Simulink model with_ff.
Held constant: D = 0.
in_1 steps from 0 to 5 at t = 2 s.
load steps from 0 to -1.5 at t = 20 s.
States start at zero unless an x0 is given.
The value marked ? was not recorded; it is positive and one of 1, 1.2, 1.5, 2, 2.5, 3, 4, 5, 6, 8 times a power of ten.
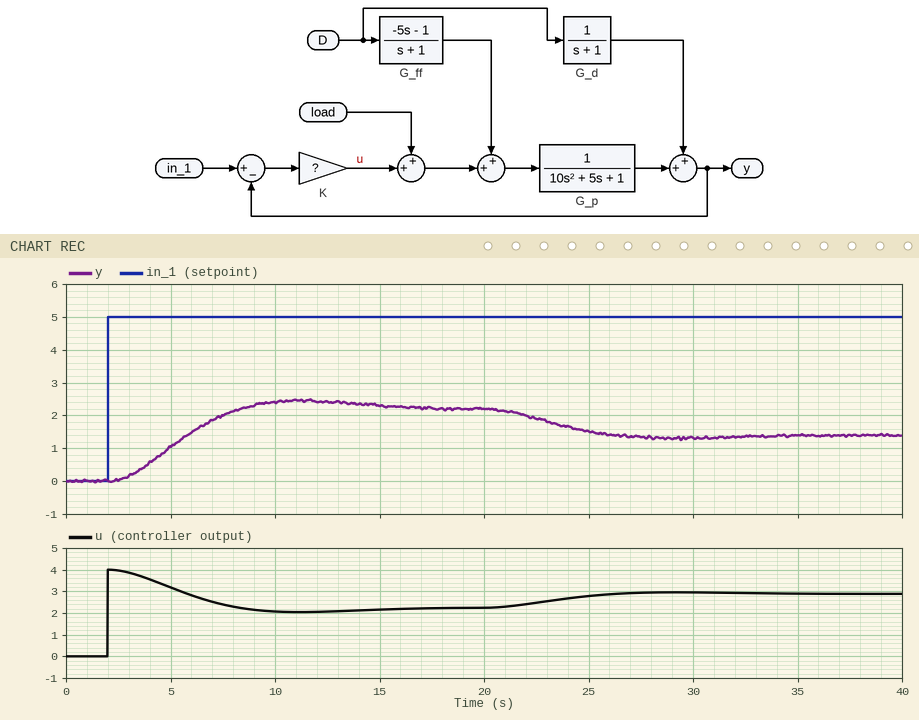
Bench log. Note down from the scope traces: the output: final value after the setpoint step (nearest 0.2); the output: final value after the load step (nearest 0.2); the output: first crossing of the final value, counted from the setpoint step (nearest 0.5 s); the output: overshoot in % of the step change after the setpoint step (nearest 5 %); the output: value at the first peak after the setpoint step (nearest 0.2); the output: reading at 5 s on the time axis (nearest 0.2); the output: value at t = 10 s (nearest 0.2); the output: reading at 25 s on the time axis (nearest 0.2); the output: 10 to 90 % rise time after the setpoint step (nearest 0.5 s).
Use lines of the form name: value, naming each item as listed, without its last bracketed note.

the output: final value after the setpoint step: 2.2
the output: final value after the load step: 1.4
the output: first crossing of the final value, counted from the setpoint step: 6.5 s
the output: overshoot in % of the step change after the setpoint step: 10 %
the output: value at the first peak after the setpoint step: 2.4
the output: reading at 5 s on the time axis: 1.0
the output: value at t = 10 s: 2.4
the output: reading at 25 s on the time axis: 1.6
the output: 10 to 90 % rise time after the setpoint step: 4.5 s
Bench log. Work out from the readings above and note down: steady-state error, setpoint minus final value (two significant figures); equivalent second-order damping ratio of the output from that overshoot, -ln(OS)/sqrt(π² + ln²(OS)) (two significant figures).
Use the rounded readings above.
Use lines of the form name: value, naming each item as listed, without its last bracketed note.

steady-state error, setpoint minus final value: 2.8
equivalent second-order damping ratio of the output from that overshoot, -ln(OS)/sqrt(π² + ln²(OS)): 0.59
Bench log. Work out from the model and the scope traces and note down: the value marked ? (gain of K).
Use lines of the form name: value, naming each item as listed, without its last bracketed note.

the value marked ?: 0.8
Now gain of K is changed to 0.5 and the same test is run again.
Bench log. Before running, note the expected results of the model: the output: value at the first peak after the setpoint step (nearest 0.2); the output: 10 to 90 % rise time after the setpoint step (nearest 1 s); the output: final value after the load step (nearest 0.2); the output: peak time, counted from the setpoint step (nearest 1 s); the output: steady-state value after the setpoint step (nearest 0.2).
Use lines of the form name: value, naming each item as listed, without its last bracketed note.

the output: value at the first peak after the setpoint step: 1.8
the output: 10 to 90 % rise time after the setpoint step: 5 s
the output: final value after the load step: 0.6
the output: peak time, counted from the setpoint step: 11 s
the output: steady-state value after the setpoint step: 1.6
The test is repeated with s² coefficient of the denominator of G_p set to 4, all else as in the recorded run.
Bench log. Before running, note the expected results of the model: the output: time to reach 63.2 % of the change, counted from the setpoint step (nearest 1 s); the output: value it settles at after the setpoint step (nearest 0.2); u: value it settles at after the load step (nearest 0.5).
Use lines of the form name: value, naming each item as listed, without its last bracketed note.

the output: time to reach 63.2 % of the change, counted from the setpoint step: 3 s
the output: value it settles at after the setpoint step: 2.2
u: value it settles at after the load step: 3.0
